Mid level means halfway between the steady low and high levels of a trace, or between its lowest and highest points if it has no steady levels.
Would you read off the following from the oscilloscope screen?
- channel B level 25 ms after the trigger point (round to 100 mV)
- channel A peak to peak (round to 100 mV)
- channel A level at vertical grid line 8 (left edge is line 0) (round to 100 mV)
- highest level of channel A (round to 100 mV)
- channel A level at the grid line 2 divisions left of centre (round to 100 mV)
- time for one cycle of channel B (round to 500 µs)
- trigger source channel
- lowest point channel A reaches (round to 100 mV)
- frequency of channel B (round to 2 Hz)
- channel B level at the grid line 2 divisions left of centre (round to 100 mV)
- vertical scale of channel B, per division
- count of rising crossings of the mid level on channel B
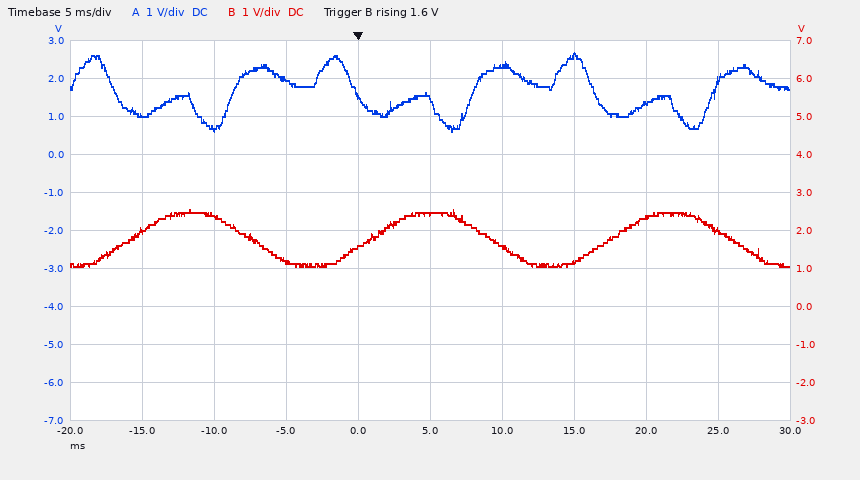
2.0 V
2.1 V
1.4 V
2.7 V
2.0 V
16.5 ms
channel B
600 mV
60 Hz
1.2 V
1 V
3
